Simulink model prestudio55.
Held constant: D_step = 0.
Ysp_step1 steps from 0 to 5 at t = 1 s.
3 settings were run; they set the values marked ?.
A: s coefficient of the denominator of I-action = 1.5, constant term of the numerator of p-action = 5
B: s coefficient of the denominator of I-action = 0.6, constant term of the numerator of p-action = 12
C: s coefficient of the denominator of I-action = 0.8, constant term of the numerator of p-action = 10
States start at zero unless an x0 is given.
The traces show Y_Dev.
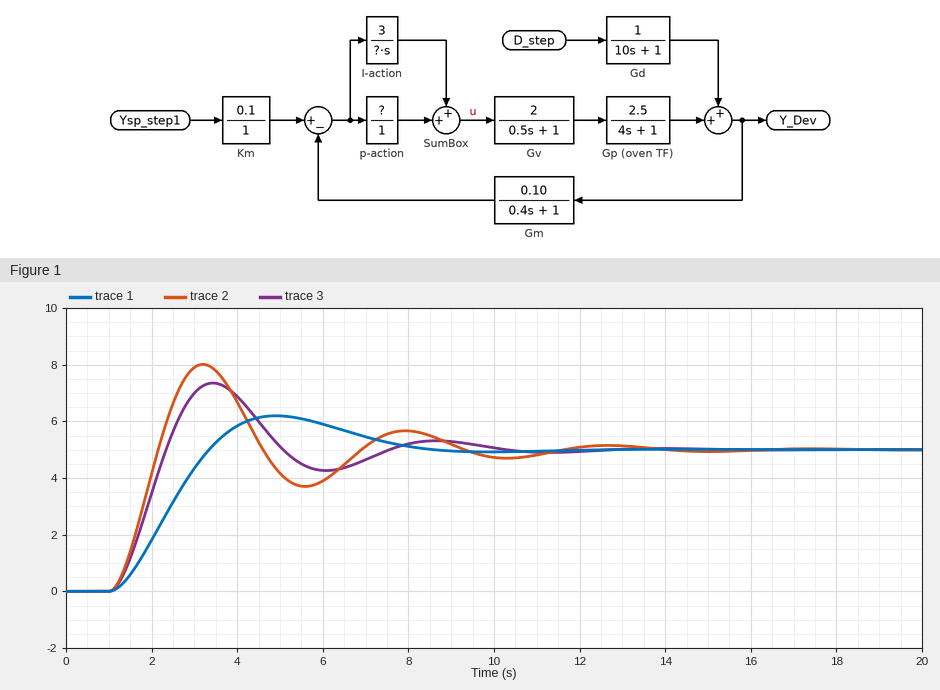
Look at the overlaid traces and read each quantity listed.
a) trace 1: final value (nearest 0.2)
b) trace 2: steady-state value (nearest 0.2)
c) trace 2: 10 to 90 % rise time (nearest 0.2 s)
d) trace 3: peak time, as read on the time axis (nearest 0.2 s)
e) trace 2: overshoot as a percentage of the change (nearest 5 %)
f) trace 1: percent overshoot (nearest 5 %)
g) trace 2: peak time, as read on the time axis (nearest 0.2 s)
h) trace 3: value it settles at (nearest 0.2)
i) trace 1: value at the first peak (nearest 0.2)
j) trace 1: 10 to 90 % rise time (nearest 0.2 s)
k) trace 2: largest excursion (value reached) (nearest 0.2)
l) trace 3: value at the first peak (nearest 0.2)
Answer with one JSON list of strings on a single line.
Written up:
["5.0", "5.0", "0.8 s", "3.4 s", "60 %", "25 %", "3.2 s", "5.0", "6.2", "1.6 s", "8.0", "7.4"]
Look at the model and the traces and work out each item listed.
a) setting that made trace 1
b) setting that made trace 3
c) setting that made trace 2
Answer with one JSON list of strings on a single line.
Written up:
["A", "C", "B"]
